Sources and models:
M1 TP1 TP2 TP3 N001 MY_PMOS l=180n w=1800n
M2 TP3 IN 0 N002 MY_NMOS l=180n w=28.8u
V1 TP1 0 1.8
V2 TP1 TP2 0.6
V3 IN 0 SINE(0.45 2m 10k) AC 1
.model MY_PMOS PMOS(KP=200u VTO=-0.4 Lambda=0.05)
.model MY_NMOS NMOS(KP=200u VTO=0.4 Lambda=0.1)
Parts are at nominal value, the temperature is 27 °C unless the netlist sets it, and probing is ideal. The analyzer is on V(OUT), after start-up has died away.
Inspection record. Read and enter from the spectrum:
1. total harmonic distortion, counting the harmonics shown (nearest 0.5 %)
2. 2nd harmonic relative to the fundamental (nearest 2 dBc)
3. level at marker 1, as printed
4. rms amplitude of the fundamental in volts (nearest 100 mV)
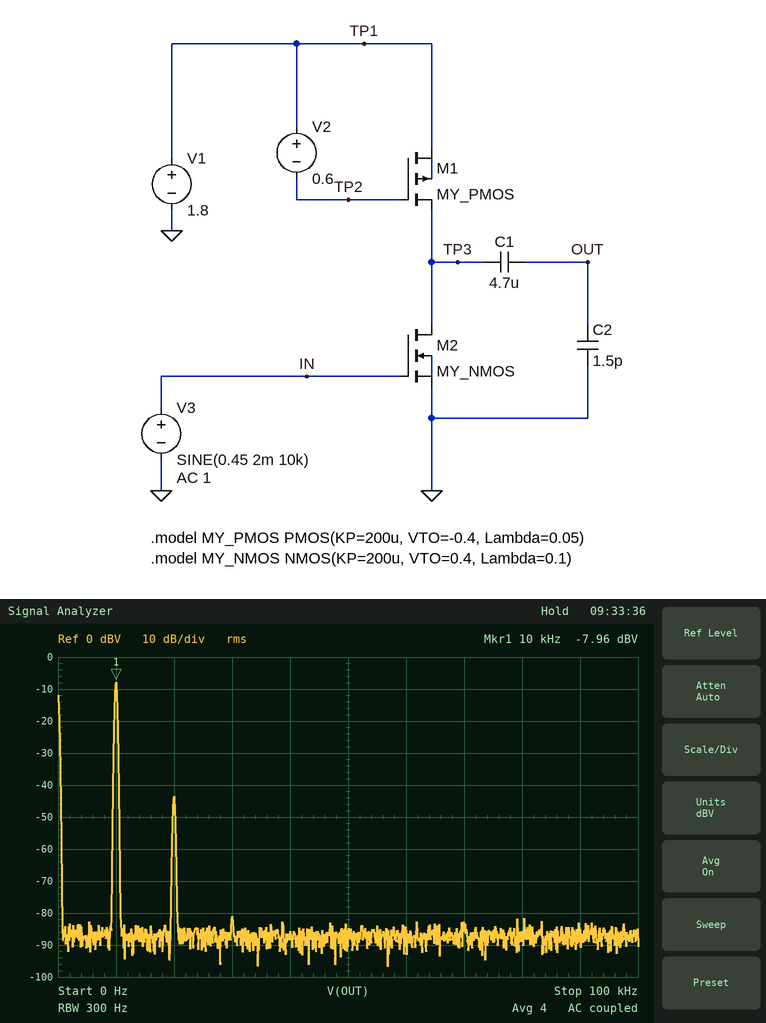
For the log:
1.5 %
-36 dBc
-7.96 dBV
400 mV
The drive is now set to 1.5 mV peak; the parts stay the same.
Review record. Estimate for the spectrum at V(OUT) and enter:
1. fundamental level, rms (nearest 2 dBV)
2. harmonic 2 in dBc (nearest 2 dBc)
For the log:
-10 dBV
-38 dBc
